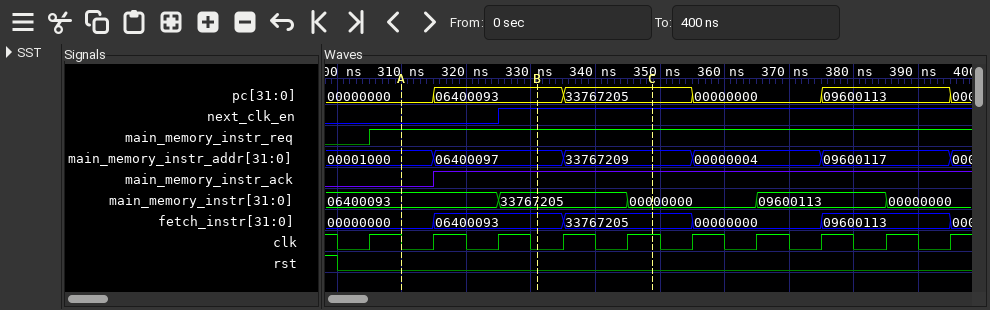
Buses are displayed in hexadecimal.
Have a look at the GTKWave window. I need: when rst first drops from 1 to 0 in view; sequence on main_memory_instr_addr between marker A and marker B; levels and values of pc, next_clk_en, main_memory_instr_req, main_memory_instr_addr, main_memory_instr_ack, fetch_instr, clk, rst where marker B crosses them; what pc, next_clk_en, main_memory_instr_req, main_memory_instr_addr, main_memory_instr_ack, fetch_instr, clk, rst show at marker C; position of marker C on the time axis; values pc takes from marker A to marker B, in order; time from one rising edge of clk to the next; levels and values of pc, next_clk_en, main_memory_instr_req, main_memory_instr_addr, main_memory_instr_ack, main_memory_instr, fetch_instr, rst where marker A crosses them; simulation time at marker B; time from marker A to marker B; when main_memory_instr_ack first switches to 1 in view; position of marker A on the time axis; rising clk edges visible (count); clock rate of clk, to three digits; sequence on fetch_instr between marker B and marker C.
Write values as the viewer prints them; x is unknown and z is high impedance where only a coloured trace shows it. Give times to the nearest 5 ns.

300 ns
00001000, 06400097
pc=06400093, next_clk_en=1, main_memory_instr_req=1, main_memory_instr_addr=06400097, main_memory_instr_ack=1, fetch_instr=06400093, clk=0, rst=0
pc=33767205, next_clk_en=1, main_memory_instr_req=1, main_memory_instr_addr=33767209, main_memory_instr_ack=1, fetch_instr=33767205, clk=1, rst=0
350 ns
00000000, 06400093
10 ns
pc=00000000, next_clk_en=0, main_memory_instr_req=1, main_memory_instr_addr=00001000, main_memory_instr_ack=0, main_memory_instr=06400093, fetch_instr=00000000, rst=0
330 ns
20 ns
315 ns
310 ns
10
100 MHz
06400093, 33767205
